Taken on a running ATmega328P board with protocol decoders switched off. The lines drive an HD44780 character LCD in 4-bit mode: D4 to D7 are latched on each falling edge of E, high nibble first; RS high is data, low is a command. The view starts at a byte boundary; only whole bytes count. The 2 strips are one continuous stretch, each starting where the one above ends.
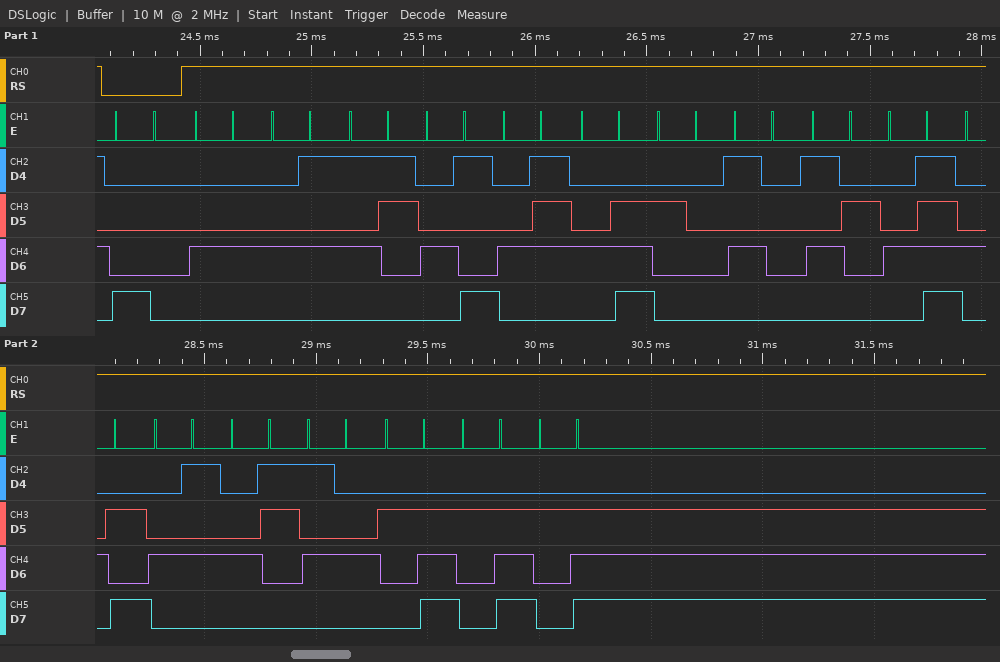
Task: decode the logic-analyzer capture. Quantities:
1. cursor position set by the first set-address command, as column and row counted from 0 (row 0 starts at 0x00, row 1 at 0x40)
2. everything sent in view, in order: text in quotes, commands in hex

column 0, row 0
0x80 "DESIGN PROJECT..."
